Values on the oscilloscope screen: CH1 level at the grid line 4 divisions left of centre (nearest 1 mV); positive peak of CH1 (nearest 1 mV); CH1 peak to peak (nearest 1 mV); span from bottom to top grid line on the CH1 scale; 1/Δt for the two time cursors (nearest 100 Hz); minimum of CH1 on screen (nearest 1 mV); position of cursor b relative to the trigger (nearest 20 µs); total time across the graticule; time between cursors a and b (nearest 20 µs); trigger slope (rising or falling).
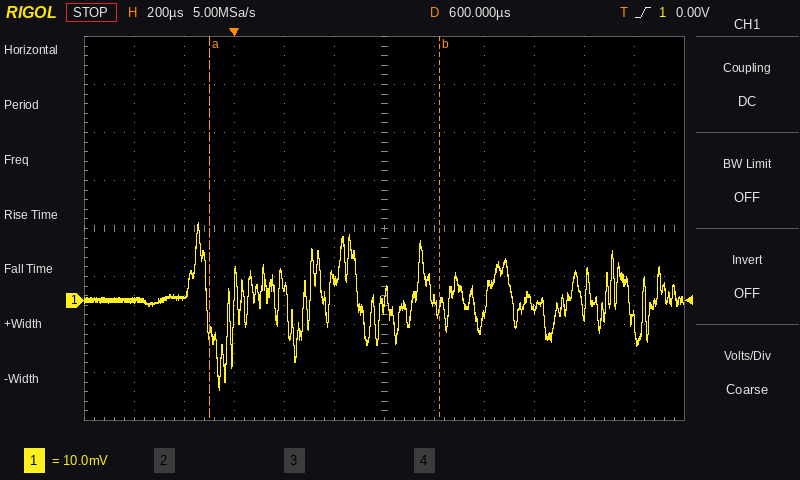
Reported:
1 mV
16 mV
35 mV
80 mV
1.1 kHz
-19 mV
+820 µs
2.4 ms
920 µs
rising
